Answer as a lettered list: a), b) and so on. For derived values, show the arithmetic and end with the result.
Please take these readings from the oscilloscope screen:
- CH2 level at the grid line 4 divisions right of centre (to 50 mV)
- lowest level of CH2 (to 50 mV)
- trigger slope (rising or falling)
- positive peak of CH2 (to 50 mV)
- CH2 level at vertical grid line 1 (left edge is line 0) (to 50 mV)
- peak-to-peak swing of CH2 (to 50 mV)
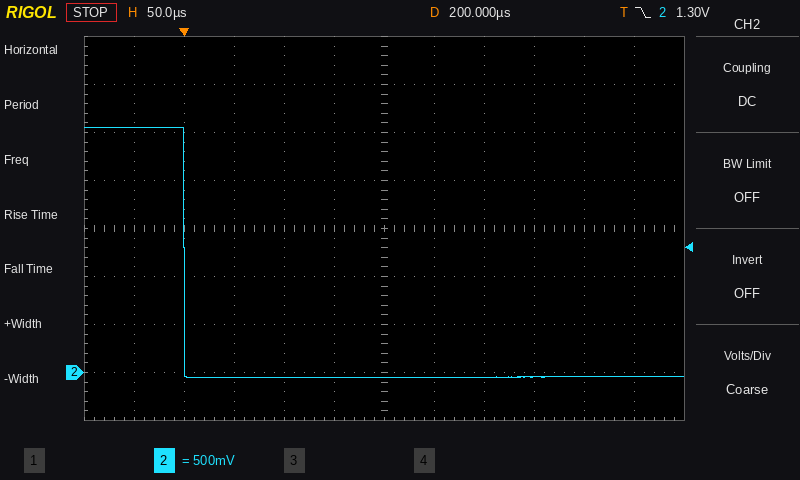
a) -50 mV
b) -50 mV
c) falling
d) 2.55 V
e) 2.55 V
f) 2.55 V − (-50 mV) = 2.60 V
